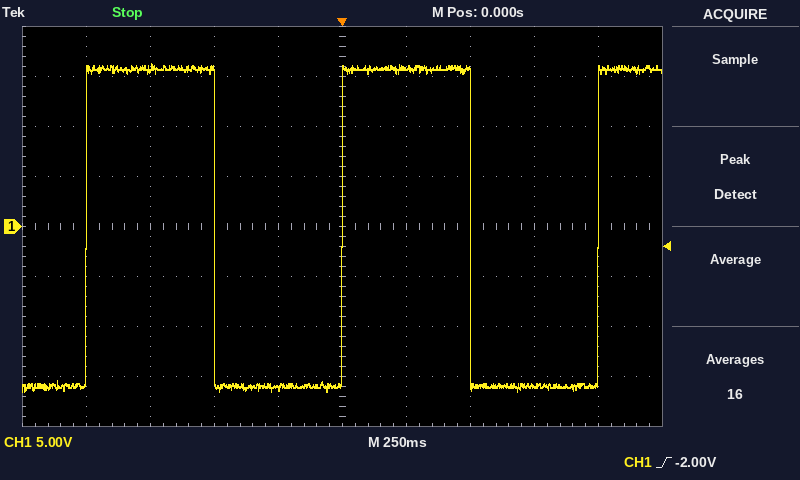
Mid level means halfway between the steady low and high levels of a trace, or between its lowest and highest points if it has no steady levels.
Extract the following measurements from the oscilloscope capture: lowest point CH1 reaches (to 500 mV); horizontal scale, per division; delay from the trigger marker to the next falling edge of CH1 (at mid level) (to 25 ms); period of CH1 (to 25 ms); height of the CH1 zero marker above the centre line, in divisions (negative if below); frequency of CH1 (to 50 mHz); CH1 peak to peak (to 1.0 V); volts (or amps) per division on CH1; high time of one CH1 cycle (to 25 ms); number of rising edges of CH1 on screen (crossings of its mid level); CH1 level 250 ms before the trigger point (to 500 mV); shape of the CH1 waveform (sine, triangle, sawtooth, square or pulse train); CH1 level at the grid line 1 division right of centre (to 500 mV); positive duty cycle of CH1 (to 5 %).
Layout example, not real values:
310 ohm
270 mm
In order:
-16.5 V
250 ms
500 ms
1.000 s
0.0 div
1.00 Hz
33.0 V
5 V
500 ms
3
-16.0 V
square
16.0 V
50 %
